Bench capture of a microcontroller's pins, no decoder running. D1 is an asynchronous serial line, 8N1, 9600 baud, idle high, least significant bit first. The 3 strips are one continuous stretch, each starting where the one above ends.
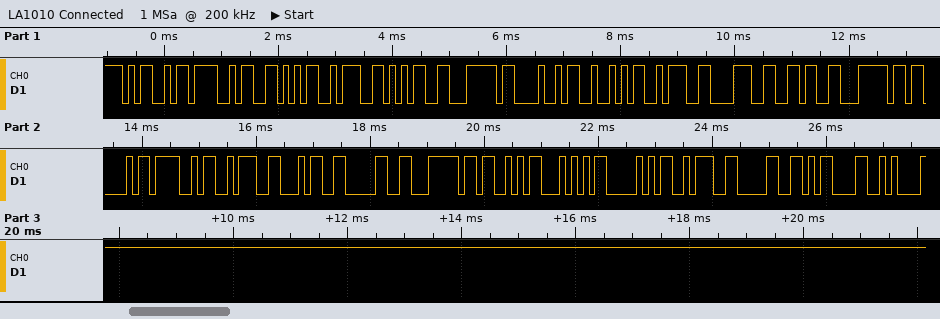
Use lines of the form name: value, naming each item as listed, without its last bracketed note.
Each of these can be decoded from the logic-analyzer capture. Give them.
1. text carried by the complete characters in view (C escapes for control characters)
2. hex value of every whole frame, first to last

text carried by the complete characters in view: "MOV:5|HR:86|CO:40|STP:0\r\n"
hex value of every whole frame, first to last: 4D 4F 56 3A 35 7C 48 52 3A 38 36 7C 43 4F 3A 34 30 7C 53 54 50 3A 30 0D 0A
